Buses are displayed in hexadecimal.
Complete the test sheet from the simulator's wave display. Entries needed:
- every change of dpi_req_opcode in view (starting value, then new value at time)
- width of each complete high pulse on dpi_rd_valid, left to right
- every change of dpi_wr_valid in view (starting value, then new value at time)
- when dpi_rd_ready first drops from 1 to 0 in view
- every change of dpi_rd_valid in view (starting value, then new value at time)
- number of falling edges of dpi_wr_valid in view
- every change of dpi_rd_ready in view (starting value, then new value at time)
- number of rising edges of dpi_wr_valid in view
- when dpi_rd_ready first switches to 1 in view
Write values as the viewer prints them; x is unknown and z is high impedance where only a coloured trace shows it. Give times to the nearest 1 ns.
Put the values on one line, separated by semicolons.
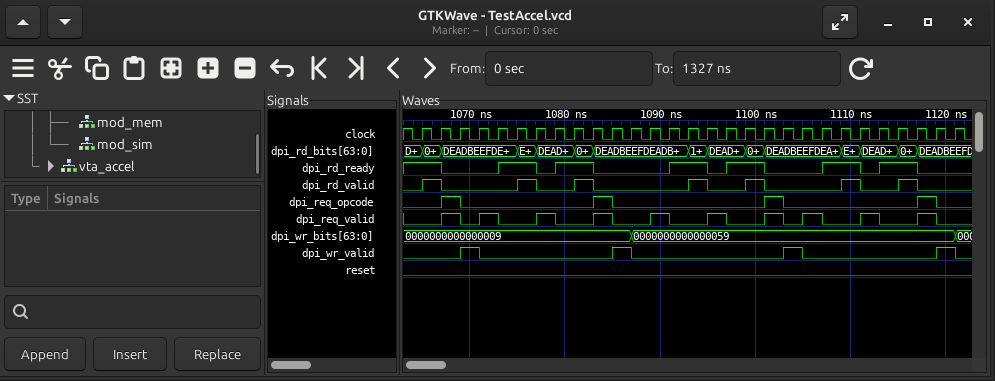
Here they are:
0, 1 at 1067 ns, 0 at 1069 ns, 1 at 1083 ns, 0 at 1085 ns, 1 at 1101 ns, 0 at 1103 ns, 1 at 1117 ns, 0 at 1119 ns; 2 ns, 2 ns, 2 ns, 2 ns, 2 ns, 2 ns, 2 ns; 0, 1 at 1069 ns, 0 at 1071 ns, 1 at 1085 ns, 0 at 1087 ns, 1 at 1103 ns, 0 at 1105 ns, 1 at 1119 ns, 0 at 1121 ns; 1067 ns; 0, 1 at 1065 ns, 0 at 1067 ns, 1 at 1075 ns, 0 at 1077 ns, 1 at 1081 ns, 0 at 1083 ns, 1 at 1093 ns, 0 at 1095 ns, 1 at 1099 ns, 0 at 1101 ns, 1 at 1109 ns, 0 at 1111 ns, 1 at 1115 ns, 0 at 1117 ns; 4; 1, 0 at 1067 ns, 1 at 1073 ns, 0 at 1077 ns, 1 at 1079 ns, 0 at 1083 ns, 1 at 1091 ns, 0 at 1095 ns, 1 at 1097 ns, 0 at 1101 ns, 1 at 1107 ns, 0 at 1111 ns, 1 at 1113 ns, 0 at 1117 ns; 4; 1073 ns
